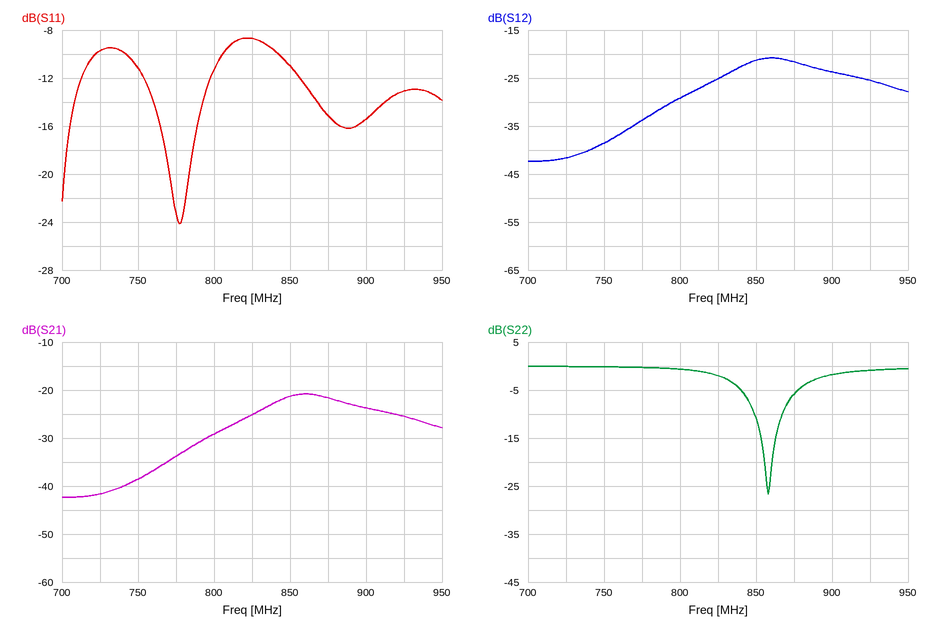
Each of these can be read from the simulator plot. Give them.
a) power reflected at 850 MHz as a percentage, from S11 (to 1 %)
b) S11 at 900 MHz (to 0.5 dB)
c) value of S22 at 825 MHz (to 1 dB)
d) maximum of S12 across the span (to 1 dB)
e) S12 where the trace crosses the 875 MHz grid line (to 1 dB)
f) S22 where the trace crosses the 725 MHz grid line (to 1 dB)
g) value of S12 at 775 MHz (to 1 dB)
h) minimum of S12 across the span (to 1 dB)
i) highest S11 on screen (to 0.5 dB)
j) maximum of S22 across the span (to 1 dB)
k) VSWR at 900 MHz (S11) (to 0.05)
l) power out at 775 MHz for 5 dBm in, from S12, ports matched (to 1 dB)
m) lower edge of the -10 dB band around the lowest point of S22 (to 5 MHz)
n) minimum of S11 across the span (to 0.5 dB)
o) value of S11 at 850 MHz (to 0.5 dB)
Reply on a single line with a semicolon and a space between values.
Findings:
8 %; -15.5 dB; -2 dB; -21 dB; -22 dB; 0 dB; -34 dB; -42 dB; -8.5 dB; 0 dB; 1.40; -29 dBm; 850 MHz; -24.0 dB; -11.0 dB
